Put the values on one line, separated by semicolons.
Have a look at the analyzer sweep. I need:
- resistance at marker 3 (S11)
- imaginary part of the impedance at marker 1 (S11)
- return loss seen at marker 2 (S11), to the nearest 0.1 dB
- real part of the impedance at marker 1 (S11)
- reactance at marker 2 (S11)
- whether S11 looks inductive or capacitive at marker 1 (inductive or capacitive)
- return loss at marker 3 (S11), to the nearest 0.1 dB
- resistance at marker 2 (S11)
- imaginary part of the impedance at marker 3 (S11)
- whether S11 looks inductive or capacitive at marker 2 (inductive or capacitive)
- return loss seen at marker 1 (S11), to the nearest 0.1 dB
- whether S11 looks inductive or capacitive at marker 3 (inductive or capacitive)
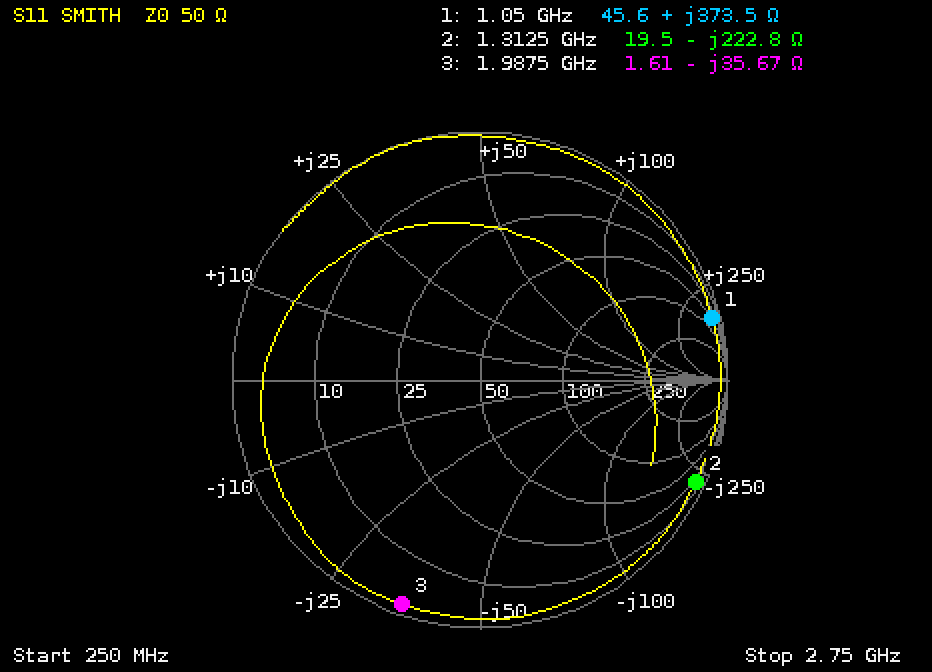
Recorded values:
1.61 Ω; +373.5 Ω; 0.3 dB; 45.6 Ω; -222.8 Ω; inductive; 0.4 dB; 19.5 Ω; -35.67 Ω; capacitive; 0.3 dB; capacitive
